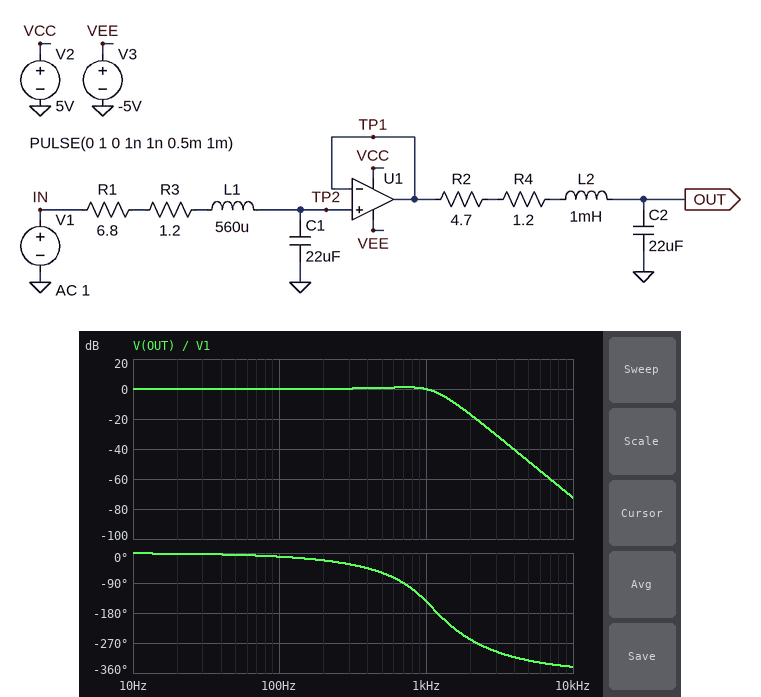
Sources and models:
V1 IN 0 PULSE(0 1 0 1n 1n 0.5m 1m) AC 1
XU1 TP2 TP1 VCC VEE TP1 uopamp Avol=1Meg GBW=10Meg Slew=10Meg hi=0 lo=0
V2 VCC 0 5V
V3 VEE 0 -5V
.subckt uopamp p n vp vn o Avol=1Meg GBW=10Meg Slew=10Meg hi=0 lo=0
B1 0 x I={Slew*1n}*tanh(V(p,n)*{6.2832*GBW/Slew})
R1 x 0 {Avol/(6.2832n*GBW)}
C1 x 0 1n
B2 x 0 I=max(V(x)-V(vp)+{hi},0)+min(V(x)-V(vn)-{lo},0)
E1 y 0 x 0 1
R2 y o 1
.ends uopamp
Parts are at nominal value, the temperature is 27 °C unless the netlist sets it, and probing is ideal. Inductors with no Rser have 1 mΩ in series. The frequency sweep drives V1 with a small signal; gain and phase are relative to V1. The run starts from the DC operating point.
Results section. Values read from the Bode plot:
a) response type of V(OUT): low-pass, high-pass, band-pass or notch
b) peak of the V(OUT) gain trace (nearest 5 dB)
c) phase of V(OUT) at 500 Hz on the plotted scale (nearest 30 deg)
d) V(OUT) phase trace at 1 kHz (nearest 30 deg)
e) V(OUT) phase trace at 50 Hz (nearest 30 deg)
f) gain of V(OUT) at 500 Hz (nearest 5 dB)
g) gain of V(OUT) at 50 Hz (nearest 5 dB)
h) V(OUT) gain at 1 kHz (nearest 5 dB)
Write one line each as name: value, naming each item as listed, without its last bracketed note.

response type of V(OUT): low-pass, high-pass, band-pass or notch: low-pass
peak of the V(OUT) gain trace: 0 dB
phase of V(OUT) at 500 Hz on the plotted scale: -60 deg
V(OUT) phase trace at 1 kHz: -150 deg
V(OUT) phase trace at 50 Hz: 0 deg
gain of V(OUT) at 500 Hz: 0 dB
gain of V(OUT) at 50 Hz: 0 dB
V(OUT) gain at 1 kHz: 0 dB
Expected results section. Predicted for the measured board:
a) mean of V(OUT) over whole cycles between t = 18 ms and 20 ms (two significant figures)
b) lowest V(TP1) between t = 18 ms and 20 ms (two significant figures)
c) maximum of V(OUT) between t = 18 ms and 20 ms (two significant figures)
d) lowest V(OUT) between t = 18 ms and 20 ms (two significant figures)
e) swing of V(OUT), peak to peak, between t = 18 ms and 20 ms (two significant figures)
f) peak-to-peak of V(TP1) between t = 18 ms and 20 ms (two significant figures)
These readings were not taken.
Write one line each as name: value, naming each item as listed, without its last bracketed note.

mean of V(OUT) over whole cycles between t = 18 ms and 20 ms: 500 mV
lowest V(TP1) between t = 18 ms and 20 ms: -12 mV
maximum of V(OUT) between t = 18 ms and 20 ms: 1.1 V
lowest V(OUT) between t = 18 ms and 20 ms: -140 mV
swing of V(OUT), peak to peak, between t = 18 ms and 20 ms: 1.3 V
peak-to-peak of V(TP1) between t = 18 ms and 20 ms: 1.0 V
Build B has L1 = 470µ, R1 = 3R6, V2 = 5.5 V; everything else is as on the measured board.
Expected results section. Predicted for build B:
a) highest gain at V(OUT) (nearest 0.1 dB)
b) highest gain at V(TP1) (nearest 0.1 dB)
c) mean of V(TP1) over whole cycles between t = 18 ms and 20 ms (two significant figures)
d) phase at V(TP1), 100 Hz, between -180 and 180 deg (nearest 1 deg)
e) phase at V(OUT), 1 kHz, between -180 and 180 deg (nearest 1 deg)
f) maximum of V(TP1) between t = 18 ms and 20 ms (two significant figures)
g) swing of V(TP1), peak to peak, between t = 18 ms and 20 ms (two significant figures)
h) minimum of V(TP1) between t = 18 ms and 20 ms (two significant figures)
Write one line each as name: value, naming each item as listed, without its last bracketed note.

highest gain at V(OUT): 3.0 dB
highest gain at V(TP1): 1.0 dB
mean of V(TP1) over whole cycles between t = 18 ms and 20 ms: 500 mV
phase at V(TP1), 100 Hz, between -180 and 180 deg: -4 deg
phase at V(OUT), 1 kHz, between -180 and 180 deg: -129 deg
maximum of V(TP1) between t = 18 ms and 20 ms: 1.2 V
swing of V(TP1), peak to peak, between t = 18 ms and 20 ms: 1.3 V
minimum of V(TP1) between t = 18 ms and 20 ms: -160 mV
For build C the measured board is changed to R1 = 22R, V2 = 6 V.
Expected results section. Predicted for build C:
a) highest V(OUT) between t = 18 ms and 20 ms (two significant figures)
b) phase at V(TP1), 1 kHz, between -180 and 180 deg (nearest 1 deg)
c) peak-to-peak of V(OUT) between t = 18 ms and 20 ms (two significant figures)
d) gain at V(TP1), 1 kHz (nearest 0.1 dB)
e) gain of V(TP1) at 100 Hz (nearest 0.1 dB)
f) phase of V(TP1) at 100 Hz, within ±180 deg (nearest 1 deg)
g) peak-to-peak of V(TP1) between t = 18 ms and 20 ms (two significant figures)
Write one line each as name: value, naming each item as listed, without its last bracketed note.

highest V(OUT) between t = 18 ms and 20 ms: 740 mV
phase at V(TP1), 1 kHz, between -180 and 180 deg: -81 deg
peak-to-peak of V(OUT) between t = 18 ms and 20 ms: 480 mV
gain at V(TP1), 1 kHz: -10.2 dB
gain of V(TP1) at 100 Hz: -0.4 dB
phase of V(TP1) at 100 Hz, within ±180 deg: -18 deg
peak-to-peak of V(TP1) between t = 18 ms and 20 ms: 450 mV
